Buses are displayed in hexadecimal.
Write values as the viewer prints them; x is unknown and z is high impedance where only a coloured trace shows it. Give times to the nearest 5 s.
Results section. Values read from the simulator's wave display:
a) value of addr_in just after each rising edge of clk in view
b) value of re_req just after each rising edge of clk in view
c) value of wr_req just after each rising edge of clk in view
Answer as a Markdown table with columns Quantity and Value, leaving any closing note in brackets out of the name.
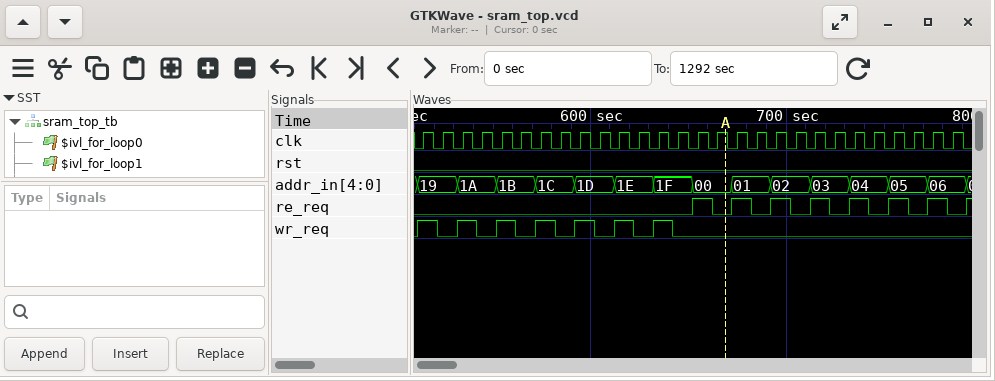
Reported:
| Quantity | Value |
|---|---|
| value of addr_in just after each rising edge of clk in view | 19, 19, 1A, 1A, 1B, 1B, 1C, 1C, 1D, 1D, 1E, 1E, 1F, 1F, 00, 00, 01, 01, 02, 02, 03, 03, 04, 04, 05, 05, 06, 06 |
| value of re_req just after each rising edge of clk in view | 0 0 0 0 0 0 0 0 0 0 0 0 0 0 1 0 1 0 1 0 1 0 1 0 1 0 1 0 |
| value of wr_req just after each rising edge of clk in view | 1 0 1 0 1 0 1 0 1 0 1 0 1 0 0 0 0 0 0 0 0 0 0 0 0 0 0 0 |
